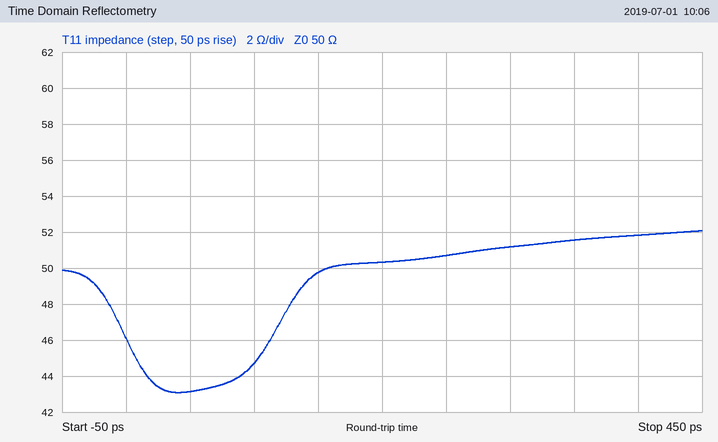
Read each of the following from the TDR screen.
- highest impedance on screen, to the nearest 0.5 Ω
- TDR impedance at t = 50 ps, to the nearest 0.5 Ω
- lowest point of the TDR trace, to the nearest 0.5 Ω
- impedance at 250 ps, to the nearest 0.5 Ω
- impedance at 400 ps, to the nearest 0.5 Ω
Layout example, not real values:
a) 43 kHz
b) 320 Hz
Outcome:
a) 52.0 Ω
b) 43.0 Ω
c) 43.0 Ω
d) 50.5 Ω
e) 52.0 Ω
